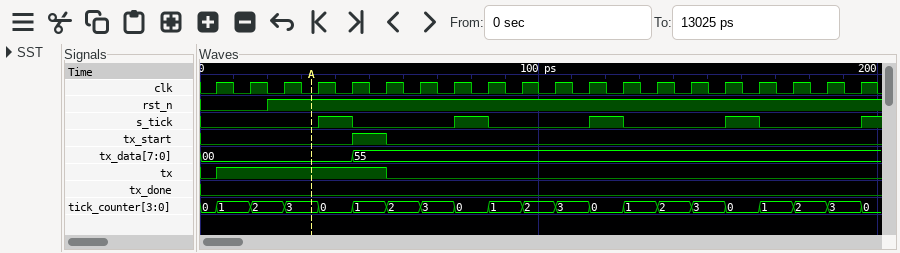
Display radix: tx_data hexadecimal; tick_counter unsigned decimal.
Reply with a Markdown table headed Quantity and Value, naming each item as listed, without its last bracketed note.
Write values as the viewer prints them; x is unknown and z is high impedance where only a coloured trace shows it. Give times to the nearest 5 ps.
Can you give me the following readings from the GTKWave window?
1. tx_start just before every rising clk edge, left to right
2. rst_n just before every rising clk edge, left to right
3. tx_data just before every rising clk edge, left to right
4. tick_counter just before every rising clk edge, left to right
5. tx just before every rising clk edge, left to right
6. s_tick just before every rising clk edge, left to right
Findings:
| Quantity | Value |
|---|---|
| tx_start just before every rising clk edge, left to right | 0 0 0 0 0 1 0 0 0 0 0 0 0 0 0 0 0 0 0 0 |
| rst_n just before every rising clk edge, left to right | 0 0 1 1 1 1 1 1 1 1 1 1 1 1 1 1 1 1 1 1 |
| tx_data just before every rising clk edge, left to right | 00, 00, 00, 00, 00, 55, 55, 55, 55, 55, 55, 55, 55, 55, 55, 55, 55, 55, 55, 55 |
| tick_counter just before every rising clk edge, left to right | 0, 1, 2, 3, 0, 1, 2, 3, 0, 1, 2, 3, 0, 1, 2, 3, 0, 1, 2, 3 |
| tx just before every rising clk edge, left to right | 0 1 1 1 1 1 0 0 0 0 0 0 0 0 0 0 0 0 0 0 |
| s_tick just before every rising clk edge, left to right | 0 0 0 0 1 0 0 0 1 0 0 0 1 0 0 0 1 0 0 0 |
